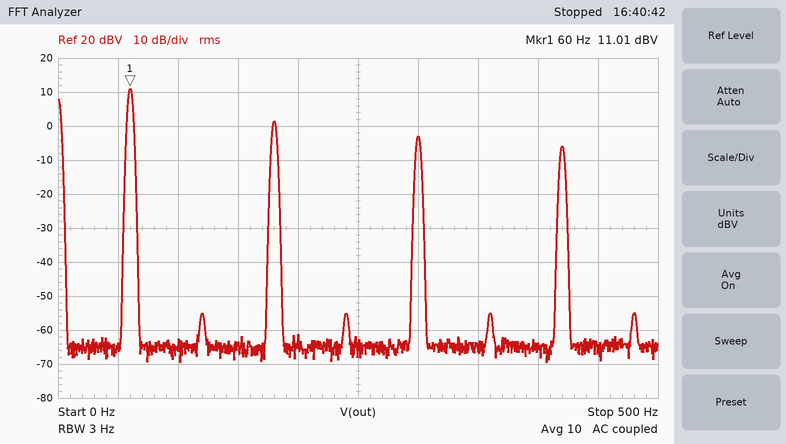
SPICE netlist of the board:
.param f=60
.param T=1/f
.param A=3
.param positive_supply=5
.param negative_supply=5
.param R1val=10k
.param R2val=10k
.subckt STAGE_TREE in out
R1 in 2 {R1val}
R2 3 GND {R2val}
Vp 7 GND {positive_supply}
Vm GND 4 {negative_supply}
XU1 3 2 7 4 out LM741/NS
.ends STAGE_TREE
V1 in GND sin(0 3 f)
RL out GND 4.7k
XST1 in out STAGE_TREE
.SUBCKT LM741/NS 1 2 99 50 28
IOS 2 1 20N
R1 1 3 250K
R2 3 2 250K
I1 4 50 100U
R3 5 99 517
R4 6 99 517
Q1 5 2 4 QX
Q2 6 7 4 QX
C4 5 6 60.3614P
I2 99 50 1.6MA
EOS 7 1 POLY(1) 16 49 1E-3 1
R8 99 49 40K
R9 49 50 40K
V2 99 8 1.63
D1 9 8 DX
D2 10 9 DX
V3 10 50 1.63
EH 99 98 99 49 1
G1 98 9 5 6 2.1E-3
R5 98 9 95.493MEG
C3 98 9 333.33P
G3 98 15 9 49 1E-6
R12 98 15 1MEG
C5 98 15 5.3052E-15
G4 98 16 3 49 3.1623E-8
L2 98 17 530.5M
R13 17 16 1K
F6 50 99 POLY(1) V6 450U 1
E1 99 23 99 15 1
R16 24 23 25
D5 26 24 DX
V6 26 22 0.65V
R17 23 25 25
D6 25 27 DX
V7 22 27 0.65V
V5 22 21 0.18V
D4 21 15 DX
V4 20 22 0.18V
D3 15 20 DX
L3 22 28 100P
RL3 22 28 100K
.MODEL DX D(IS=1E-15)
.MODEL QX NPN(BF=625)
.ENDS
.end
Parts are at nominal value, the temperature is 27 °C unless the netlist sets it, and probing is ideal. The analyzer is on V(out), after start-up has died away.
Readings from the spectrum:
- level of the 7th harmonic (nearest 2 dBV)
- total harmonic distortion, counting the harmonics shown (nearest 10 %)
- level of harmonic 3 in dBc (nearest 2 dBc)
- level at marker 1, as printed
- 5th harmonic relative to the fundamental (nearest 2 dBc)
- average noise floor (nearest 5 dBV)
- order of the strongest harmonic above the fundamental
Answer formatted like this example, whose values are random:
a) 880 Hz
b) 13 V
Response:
a) -6 dBV
b) 40 %
c) -10 dBc
d) 11.01 dBV
e) -14 dBc
f) -65 dBV
g) 3
